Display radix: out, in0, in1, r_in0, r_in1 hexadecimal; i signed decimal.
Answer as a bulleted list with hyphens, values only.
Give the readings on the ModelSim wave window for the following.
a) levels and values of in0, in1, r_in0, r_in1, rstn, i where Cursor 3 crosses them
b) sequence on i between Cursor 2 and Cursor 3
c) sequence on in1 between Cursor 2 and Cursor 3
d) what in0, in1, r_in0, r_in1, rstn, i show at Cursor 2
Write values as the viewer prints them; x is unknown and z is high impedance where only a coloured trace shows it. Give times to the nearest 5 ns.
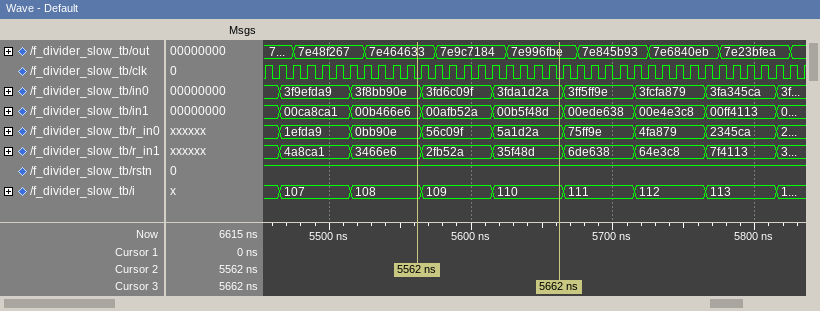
- in0=3fda1d2a, in1=00b5f48d, r_in0=5a1d2a, r_in1=35f48d, rstn=1, i=110
- 108, 109, 110
- 00b466e6, 00afb52a, 00b5f48d
- in0=3f8bb90e, in1=00b466e6, r_in0=0bb90e, r_in1=3466e6, rstn=1, i=108
